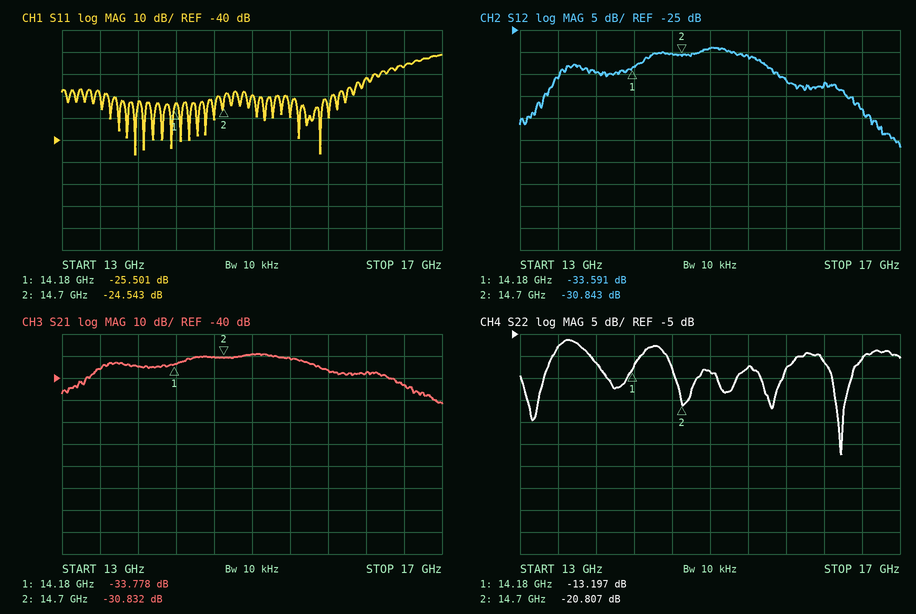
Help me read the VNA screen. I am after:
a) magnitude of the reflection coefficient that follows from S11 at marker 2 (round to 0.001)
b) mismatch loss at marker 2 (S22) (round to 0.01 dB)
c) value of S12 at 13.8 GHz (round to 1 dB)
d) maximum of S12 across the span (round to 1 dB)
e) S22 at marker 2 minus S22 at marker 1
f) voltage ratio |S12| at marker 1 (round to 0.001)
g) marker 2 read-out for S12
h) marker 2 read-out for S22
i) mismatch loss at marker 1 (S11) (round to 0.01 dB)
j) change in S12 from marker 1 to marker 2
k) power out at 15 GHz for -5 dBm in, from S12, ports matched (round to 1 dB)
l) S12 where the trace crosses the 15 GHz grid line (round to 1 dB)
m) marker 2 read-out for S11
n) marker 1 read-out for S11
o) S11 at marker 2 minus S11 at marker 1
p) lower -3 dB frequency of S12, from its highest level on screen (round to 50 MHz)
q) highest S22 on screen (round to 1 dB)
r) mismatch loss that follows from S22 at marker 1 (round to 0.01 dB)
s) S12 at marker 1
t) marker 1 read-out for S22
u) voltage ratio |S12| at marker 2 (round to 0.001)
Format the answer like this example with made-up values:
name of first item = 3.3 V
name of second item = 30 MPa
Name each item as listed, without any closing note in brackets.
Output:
magnitude of the reflection coefficient that follows from S11 at marker 2 = 0.059
mismatch loss at marker 2 (S22) = 0.04 dB
value of S12 at 13.8 GHz = -35 dB
maximum of S12 across the span = -29 dB
S22 at marker 2 minus S22 at marker 1 = -7.610 dB
voltage ratio |S12| at marker 1 = 0.021
marker 2 read-out for S12 = -30.843 dB
marker 2 read-out for S22 = -20.807 dB
mismatch loss at marker 1 (S11) = 0.01 dB
change in S12 from marker 1 to marker 2 = 2.748 dB
power out at 15 GHz for -5 dBm in, from S12, ports matched = -34 dBm
S12 where the trace crosses the 15 GHz grid line = -29 dB
marker 2 read-out for S11 = -24.543 dB
marker 1 read-out for S11 = -25.501 dB
S11 at marker 2 minus S11 at marker 1 = 0.958 dB
lower -3 dB frequency of S12, from its highest level on screen = 14.30 GHz
highest S22 on screen = -6 dB
mismatch loss that follows from S22 at marker 1 = 0.21 dB
S12 at marker 1 = -33.591 dB
marker 1 read-out for S22 = -13.197 dB
voltage ratio |S12| at marker 2 = 0.029
